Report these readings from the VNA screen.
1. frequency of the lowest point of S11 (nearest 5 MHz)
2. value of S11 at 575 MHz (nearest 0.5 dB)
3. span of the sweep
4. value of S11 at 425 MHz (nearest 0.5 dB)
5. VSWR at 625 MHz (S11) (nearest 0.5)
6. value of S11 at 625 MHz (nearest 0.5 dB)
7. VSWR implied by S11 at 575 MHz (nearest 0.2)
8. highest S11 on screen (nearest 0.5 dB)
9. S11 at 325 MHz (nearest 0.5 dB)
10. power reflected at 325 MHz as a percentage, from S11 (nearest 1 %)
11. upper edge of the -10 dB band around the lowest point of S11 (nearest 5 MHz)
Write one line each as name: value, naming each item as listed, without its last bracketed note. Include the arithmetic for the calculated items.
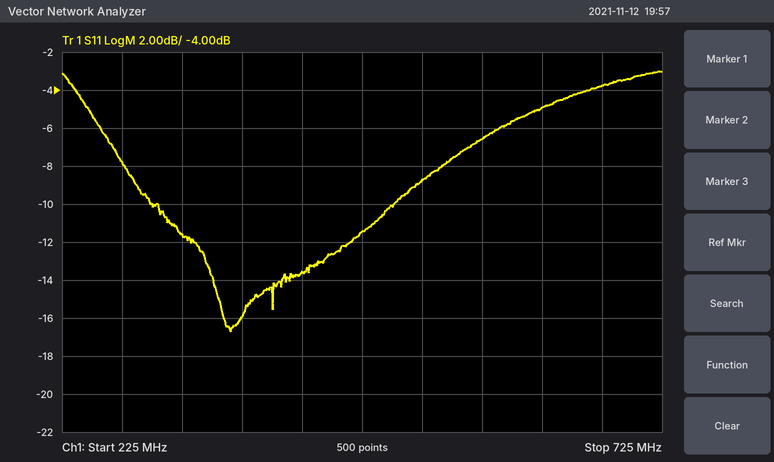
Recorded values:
frequency of the lowest point of S11: 365 MHz
value of S11 at 575 MHz: -6.5 dB
span of the sweep: 500 MHz
value of S11 at 425 MHz: -13.5 dB
VSWR at 625 MHz (S11): |Γ| = 10^(-5/20) = 0.5623; VSWR = (1 + 0.5623)/(1 − 0.5623) ≈ 3.57, so 3.5 to the nearest 0.5
value of S11 at 625 MHz: -5.0 dB
VSWR implied by S11 at 575 MHz: |Γ| = 10^(-6.5/20) = 0.4732; VSWR = (1 + 0.4732)/(1 − 0.4732) ≈ 2.8
highest S11 on screen: -3.0 dB
S11 at 325 MHz: -11.5 dB
power reflected at 325 MHz as a percentage, from S11: 10^(-11.5/10) ≈ 7 %
upper edge of the -10 dB band around the lowest point of S11: 500 MHz
